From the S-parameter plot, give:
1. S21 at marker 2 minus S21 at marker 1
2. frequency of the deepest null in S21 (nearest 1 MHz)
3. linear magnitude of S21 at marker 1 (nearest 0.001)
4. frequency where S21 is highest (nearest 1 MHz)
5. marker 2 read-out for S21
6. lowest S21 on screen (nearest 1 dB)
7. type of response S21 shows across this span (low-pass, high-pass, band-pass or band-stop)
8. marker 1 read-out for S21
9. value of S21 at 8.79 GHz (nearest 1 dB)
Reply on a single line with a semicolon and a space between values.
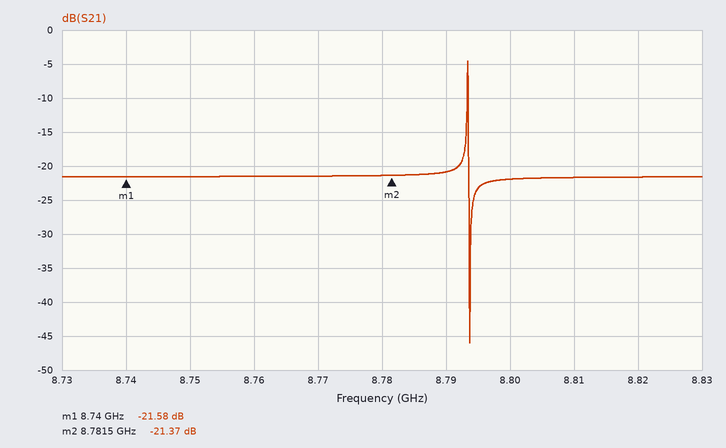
0.21 dB; 8.794 GHz; 0.083; 8.793 GHz; -21.37 dB; -46 dB; band-pass; -21.58 dB; -21 dB
